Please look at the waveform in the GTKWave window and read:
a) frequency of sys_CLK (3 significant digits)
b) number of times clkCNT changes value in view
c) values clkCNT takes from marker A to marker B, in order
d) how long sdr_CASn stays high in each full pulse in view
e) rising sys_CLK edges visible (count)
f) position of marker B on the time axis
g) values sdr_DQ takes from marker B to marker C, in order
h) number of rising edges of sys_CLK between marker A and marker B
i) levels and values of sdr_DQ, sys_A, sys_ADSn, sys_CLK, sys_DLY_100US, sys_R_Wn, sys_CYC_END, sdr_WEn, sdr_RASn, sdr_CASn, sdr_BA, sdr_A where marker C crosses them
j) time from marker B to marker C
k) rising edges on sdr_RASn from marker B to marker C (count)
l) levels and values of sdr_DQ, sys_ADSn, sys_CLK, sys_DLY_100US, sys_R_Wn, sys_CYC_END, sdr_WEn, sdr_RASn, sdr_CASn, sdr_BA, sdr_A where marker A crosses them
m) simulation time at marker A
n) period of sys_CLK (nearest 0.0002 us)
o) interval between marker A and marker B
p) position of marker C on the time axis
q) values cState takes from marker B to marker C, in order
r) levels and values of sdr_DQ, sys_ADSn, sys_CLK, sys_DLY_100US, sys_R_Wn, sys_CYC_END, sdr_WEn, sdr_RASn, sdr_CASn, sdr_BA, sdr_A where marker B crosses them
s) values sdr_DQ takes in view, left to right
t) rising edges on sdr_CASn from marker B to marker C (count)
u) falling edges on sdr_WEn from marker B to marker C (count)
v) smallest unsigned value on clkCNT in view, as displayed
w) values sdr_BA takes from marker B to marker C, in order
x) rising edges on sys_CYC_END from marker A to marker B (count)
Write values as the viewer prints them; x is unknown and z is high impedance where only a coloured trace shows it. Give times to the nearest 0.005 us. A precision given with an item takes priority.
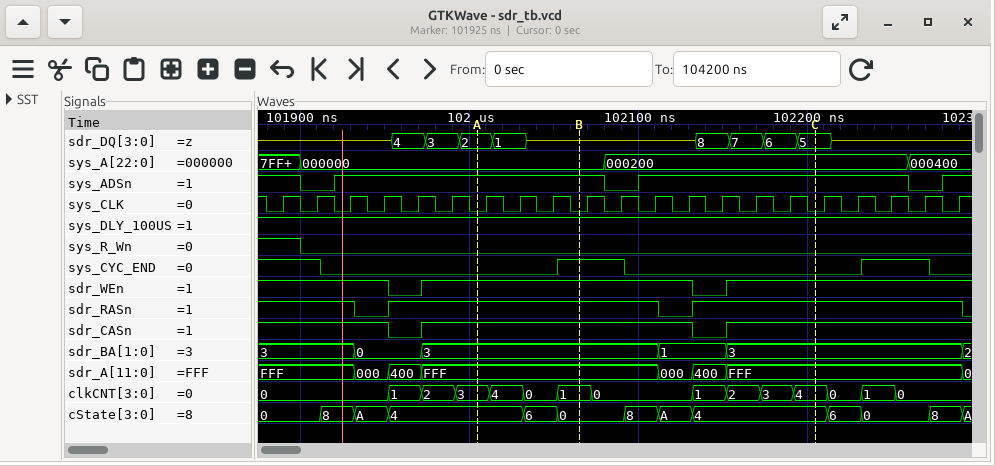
50.0 MHz
14
3, 4, 0, 1
0.16 us
21
102.065 us
z, 8, 7, 6, 5
3
sdr_DQ=5, sys_A=000200, sys_ADSn=1, sys_CLK=0, sys_DLY_100US=1, sys_R_Wn=0, sys_CYC_END=0, sdr_WEn=1, sdr_RASn=1, sdr_CASn=1, sdr_BA=3, sdr_A=FFF
0.14 us
1
sdr_DQ=2, sys_ADSn=1, sys_CLK=0, sys_DLY_100US=1, sys_R_Wn=0, sys_CYC_END=0, sdr_WEn=1, sdr_RASn=1, sdr_CASn=1, sdr_BA=3, sdr_A=FFF
102.005 us
0.02 us
0.06 us
102.205 us
0, 8, A, 4
sdr_DQ=z, sys_ADSn=1, sys_CLK=0, sys_DLY_100US=1, sys_R_Wn=0, sys_CYC_END=1, sdr_WEn=1, sdr_RASn=1, sdr_CASn=1, sdr_BA=3, sdr_A=FFF
z, 4, 3, 2, 1, z, 8, 7, 6, 5, z
1
1
0
3, 1, 3
1
